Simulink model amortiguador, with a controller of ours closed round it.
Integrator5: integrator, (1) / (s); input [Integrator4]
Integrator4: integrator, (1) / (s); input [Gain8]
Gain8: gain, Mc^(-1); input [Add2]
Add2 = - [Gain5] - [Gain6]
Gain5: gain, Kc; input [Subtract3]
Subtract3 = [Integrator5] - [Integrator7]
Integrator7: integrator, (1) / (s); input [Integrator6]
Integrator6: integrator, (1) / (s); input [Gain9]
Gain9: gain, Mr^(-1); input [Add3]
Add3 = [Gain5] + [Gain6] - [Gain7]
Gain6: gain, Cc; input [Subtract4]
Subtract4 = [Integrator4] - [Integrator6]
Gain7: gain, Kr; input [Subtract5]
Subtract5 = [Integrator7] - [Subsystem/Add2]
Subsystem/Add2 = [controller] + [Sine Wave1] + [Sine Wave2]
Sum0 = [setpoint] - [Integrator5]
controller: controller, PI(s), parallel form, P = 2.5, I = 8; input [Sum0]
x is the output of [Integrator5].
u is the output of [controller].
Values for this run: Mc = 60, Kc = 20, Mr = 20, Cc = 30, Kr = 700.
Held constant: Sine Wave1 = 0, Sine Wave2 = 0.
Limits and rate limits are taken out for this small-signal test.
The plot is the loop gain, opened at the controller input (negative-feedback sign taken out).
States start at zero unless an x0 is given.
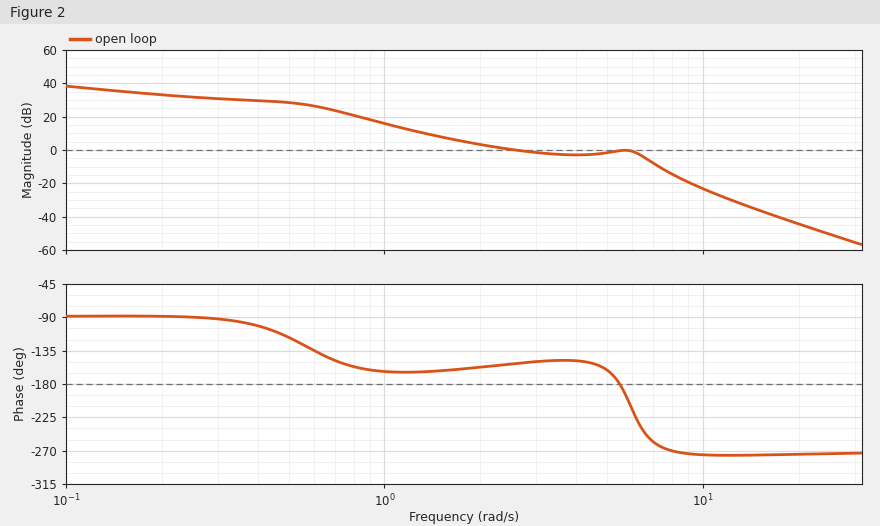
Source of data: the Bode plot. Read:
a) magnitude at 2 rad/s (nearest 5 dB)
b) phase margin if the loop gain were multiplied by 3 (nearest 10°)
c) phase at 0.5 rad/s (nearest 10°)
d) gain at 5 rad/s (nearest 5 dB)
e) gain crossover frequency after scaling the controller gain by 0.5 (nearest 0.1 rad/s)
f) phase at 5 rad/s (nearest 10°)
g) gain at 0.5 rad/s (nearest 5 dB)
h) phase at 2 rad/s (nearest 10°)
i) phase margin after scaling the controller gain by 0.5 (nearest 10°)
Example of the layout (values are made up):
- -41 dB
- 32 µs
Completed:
- 5 dB
- -80°
- -120°
- 0 dB
- 1.7 rad/s
- -160°
- 30 dB
- -160°
- 20°
